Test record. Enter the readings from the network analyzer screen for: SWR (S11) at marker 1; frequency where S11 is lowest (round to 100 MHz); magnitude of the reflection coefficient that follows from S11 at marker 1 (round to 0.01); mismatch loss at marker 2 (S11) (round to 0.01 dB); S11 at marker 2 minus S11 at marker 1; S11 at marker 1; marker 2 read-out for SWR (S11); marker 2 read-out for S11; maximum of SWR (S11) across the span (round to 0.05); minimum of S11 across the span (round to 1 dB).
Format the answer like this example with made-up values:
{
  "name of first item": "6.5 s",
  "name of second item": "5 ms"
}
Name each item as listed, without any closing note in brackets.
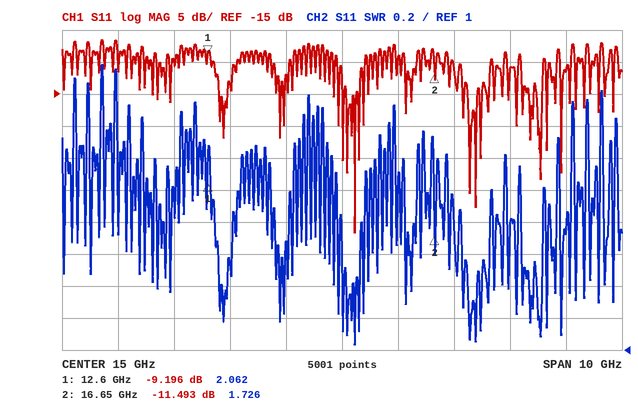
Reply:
{
  "SWR (S11) at marker 1": "2.062",
  "frequency where S11 is lowest": "15.2 GHz",
  "magnitude of the reflection coefficient that follows from S11 at marker 1": "0.35",
  "mismatch loss at marker 2 (S11)": "0.32 dB",
  "S11 at marker 2 minus S11 at marker 1": "-2.297 dB",
  "S11 at marker 1": "-9.196 dB",
  "marker 2 read-out for SWR": "1.726",
  "marker 2 read-out for S11": "-11.493 dB",
  "maximum of SWR (S11) across the span": "2.80",
  "minimum of S11 across the span": "-37 dB"
}
